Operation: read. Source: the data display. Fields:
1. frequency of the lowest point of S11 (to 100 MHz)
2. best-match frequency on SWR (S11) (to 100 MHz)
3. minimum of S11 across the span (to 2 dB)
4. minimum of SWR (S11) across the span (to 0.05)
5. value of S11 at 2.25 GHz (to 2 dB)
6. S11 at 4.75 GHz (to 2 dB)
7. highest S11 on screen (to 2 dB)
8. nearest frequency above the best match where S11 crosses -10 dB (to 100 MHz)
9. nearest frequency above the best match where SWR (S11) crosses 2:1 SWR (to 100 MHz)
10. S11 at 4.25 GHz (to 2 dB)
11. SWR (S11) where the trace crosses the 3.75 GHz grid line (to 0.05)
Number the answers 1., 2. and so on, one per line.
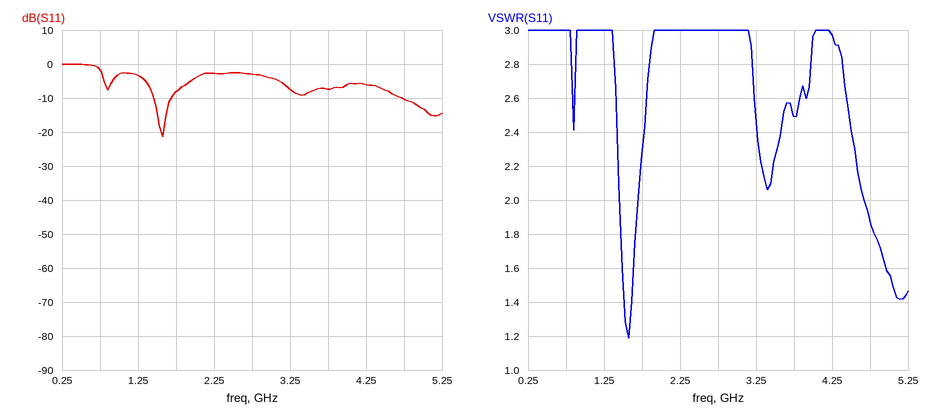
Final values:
1. 1.6 GHz
2. 1.6 GHz
3. -22 dB
4. 1.20
5. -2 dB
6. -10 dB
7. 0 dB
8. 1.7 GHz
9. 1.7 GHz
10. -6 dB
11. 2.50
